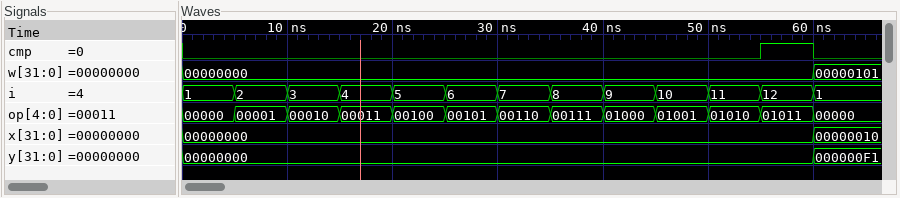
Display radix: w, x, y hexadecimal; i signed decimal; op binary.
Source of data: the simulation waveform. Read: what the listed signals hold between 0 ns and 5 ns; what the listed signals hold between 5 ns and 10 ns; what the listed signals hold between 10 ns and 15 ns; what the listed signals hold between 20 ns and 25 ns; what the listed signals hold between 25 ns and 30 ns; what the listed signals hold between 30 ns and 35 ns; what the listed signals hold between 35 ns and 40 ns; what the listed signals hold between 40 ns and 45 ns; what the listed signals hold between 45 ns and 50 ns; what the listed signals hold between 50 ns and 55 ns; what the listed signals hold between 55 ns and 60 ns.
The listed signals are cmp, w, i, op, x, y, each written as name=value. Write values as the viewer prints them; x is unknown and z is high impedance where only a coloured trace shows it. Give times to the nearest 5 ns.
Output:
cmp=0, w=00000000, i=1, op=00000, x=00000000, y=00000000
cmp=0, w=00000000, i=2, op=00001, x=00000000, y=00000000
cmp=0, w=00000000, i=3, op=00010, x=00000000, y=00000000
cmp=0, w=00000000, i=5, op=00100, x=00000000, y=00000000
cmp=0, w=00000000, i=6, op=00101, x=00000000, y=00000000
cmp=0, w=00000000, i=7, op=00110, x=00000000, y=00000000
cmp=0, w=00000000, i=8, op=00111, x=00000000, y=00000000
cmp=0, w=00000000, i=9, op=01000, x=00000000, y=00000000
cmp=0, w=00000000, i=10, op=01001, x=00000000, y=00000000
cmp=0, w=00000000, i=11, op=01010, x=00000000, y=00000000
cmp=1, w=00000000, i=12, op=01011, x=00000000, y=00000000
